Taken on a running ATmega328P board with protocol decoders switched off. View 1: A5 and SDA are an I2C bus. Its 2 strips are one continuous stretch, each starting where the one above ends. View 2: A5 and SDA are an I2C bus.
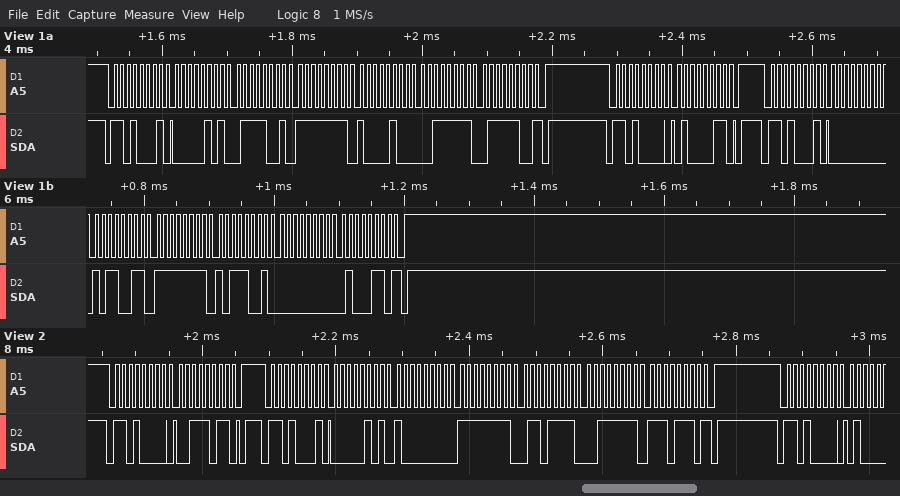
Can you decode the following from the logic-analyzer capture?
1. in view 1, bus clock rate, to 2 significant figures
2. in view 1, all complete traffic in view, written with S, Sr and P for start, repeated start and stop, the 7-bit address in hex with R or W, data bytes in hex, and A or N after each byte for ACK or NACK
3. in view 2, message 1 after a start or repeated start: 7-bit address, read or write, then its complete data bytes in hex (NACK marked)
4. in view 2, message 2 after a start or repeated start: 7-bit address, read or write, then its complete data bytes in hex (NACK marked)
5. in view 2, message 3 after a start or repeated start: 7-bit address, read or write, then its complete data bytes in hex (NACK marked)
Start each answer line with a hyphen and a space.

- 100 kHz
- S 68R A 05 A 79 A FF A 84 A 3F A 7C N P S 68W A 43 A P S 68R A 00 A B3 A FF A B9 A 00 A 46 N P
- 0x68 write: 3B
- 0x68 read: 05 80 FF 6F 3F EE NACK
- 0x68 write
